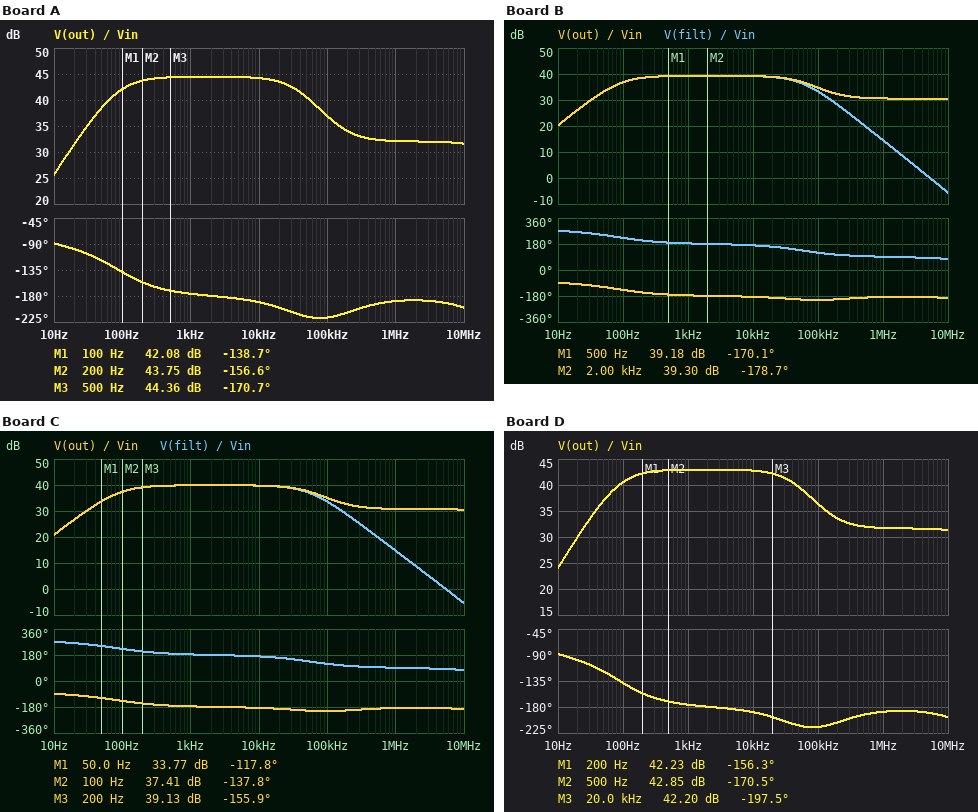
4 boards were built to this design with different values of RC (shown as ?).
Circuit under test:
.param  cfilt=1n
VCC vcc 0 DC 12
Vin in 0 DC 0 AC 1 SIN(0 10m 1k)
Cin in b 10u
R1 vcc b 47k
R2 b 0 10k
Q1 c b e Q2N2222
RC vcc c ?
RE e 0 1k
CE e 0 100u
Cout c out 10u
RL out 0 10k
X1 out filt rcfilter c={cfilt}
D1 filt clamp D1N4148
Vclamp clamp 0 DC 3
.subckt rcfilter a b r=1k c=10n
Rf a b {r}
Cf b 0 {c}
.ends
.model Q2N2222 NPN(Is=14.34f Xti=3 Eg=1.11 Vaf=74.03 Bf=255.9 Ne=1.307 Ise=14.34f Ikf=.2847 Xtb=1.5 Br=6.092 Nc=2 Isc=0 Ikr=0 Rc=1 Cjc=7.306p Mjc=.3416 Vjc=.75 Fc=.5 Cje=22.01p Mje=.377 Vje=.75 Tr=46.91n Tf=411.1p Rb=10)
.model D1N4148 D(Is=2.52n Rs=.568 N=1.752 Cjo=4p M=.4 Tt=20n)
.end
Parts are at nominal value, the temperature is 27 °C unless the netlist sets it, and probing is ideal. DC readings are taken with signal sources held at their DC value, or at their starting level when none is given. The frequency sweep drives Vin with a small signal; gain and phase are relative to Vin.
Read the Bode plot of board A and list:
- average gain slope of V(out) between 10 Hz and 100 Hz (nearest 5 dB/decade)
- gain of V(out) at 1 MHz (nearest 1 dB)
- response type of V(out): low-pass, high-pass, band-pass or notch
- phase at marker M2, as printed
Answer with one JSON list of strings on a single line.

["15 dB/decade", "32 dB", "band-pass", "-156.6 deg"]
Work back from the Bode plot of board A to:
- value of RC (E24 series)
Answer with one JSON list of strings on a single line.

["5.1 kΩ"]
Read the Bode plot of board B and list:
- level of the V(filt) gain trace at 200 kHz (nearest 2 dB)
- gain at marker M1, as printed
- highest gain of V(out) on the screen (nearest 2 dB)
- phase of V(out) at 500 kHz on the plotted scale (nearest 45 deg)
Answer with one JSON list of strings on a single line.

["28 dB", "39.18 dB", "40 dB", "-180 deg"]
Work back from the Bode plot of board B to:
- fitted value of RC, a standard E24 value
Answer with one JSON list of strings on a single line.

["2.2 kΩ"]
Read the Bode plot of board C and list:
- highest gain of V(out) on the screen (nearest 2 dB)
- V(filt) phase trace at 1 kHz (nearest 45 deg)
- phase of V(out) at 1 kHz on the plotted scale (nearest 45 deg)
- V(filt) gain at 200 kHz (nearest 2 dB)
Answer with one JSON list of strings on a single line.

["40 dB", "180 deg", "-180 deg", "28 dB"]
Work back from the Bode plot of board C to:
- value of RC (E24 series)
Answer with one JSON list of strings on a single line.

["2.4 kΩ"]
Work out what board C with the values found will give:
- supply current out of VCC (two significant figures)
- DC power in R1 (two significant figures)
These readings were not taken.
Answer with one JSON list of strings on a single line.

["1.6 mA", "2.1 mW"]
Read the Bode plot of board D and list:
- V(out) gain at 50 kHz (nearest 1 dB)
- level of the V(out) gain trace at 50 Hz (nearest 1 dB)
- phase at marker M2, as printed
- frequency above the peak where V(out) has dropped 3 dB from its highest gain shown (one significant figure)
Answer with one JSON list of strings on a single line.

["40 dB", "37 dB", "-170.5 deg", "50 kHz"]
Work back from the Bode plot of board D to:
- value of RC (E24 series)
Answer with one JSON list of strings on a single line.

["3.9 kΩ"]
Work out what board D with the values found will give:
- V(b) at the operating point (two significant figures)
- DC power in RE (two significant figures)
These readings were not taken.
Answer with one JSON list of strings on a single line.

["2.0 V", "1.9 mW"]
